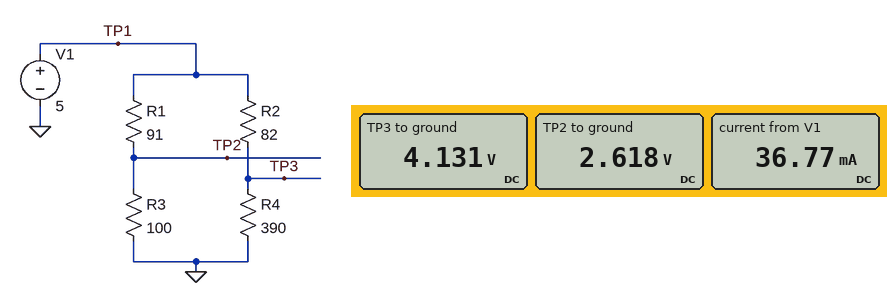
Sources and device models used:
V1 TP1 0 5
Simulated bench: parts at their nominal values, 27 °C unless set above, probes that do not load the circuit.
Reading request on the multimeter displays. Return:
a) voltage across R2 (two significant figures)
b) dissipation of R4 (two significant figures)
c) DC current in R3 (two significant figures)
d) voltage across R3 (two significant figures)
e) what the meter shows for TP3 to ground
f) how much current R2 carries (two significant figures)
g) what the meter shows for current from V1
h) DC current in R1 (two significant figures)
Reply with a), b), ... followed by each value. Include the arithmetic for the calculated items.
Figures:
a) 5 V - 4.131 V = 870 mV
b) (4.131 V)^2 / 390 Ω = 44 mW
c) (2.618 V) / 100 Ω = 26 mA
d) 2.618 V = 2.6 V
e) 4.131 V
f) (5 V - 4.131 V) / 82 Ω = 11 mA
g) 36.77 mA
h) (5 V - 2.618 V) / 91 Ω = 26 mA
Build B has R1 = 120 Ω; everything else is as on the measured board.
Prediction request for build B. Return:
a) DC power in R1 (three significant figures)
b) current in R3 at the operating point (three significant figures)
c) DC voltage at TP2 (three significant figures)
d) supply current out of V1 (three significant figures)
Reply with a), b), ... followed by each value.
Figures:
a) 62.0 mW
b) 22.7 mA
c) 2.27 V
d) 33.3 mA
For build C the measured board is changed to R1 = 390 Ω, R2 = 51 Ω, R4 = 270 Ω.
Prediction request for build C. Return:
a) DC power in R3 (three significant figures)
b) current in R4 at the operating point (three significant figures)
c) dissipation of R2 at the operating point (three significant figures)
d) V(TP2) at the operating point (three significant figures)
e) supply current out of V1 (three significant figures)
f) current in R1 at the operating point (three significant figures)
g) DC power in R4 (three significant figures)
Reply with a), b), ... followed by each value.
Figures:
a) 10.4 mW
b) 15.6 mA
c) 12.4 mW
d) 1.02 V
e) 25.8 mA
f) 10.2 mA
g) 65.5 mW
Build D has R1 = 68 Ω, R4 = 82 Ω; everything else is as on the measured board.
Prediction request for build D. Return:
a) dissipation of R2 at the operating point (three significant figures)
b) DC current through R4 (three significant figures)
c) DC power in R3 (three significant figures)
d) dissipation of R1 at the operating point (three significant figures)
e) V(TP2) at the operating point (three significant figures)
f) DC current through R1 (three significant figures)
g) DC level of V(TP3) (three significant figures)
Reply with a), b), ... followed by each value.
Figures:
a) 76.2 mW
b) 30.5 mA
c) 88.6 mW
d) 60.2 mW
e) 2.98 V
f) 29.8 mA
g) 2.50 V
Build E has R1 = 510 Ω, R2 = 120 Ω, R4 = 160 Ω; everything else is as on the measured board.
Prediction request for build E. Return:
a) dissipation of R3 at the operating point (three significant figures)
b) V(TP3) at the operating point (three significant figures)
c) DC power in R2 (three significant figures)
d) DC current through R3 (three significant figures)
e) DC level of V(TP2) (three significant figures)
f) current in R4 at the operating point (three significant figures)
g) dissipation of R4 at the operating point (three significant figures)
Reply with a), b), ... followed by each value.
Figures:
a) 6.72 mW
b) 2.86 V
c) 38.3 mW
d) 8.20 mA
e) 820 mV
f) 17.9 mA
g) 51.0 mW
